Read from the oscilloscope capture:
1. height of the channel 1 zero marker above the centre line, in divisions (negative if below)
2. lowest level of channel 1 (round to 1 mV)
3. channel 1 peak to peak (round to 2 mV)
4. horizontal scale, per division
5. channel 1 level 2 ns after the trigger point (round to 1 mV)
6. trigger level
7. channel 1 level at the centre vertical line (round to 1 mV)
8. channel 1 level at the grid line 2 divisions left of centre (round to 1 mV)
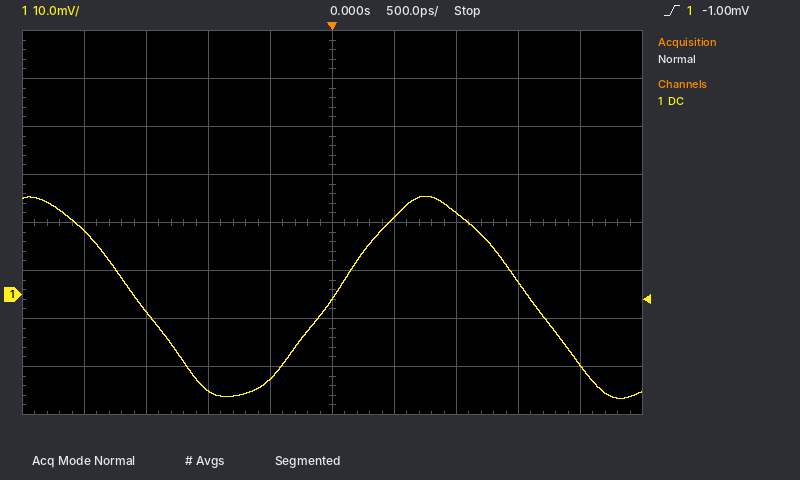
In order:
-1.5 div
-22 mV
42 mV
500 ps
-15 mV
-1.00 mV
-1 mV
-20 mV
